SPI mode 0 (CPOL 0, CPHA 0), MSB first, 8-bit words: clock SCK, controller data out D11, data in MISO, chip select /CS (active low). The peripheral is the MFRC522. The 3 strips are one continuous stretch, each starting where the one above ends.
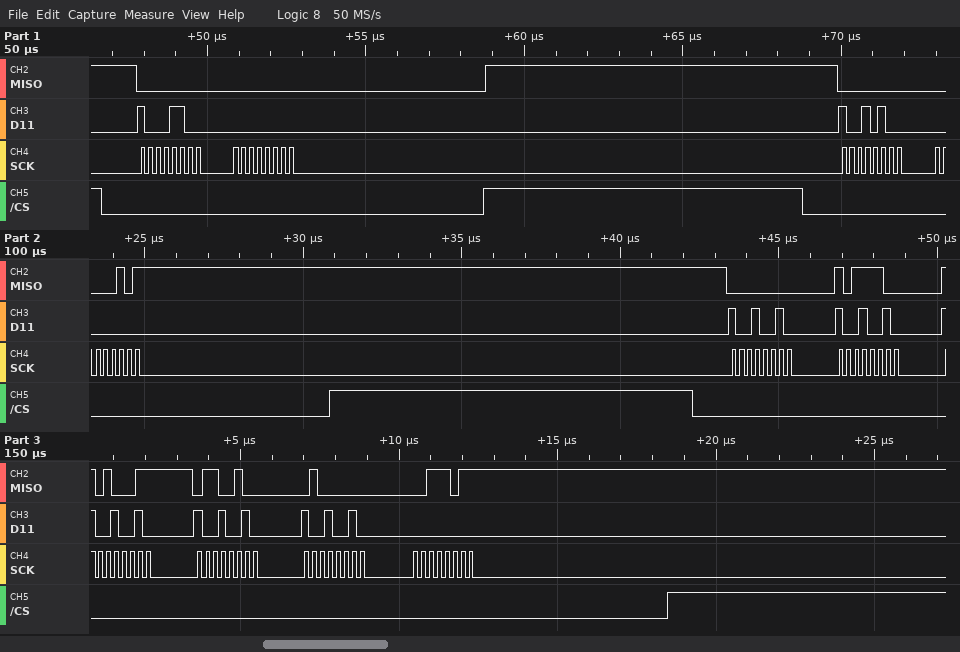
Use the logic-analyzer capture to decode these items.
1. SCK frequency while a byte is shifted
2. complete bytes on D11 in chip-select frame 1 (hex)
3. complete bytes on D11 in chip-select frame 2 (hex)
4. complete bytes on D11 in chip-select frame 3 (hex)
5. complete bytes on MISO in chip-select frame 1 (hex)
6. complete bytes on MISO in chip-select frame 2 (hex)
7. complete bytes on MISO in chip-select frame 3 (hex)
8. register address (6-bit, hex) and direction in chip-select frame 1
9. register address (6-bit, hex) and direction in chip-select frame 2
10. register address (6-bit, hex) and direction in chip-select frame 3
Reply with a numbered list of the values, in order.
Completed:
1. 4 MHz
2. 0x8C 0x00
3. 0x94 0x00
4. 0x92 0x92 0x92 0x92 0x92 0x00
5. 0x00 0x00
6. 0x00 0x05
7. 0x00 0xBC 0xA3 0x64 0x40 0x3B
8. 0x06 read
9. 0x0A read
10. 0x09 read
